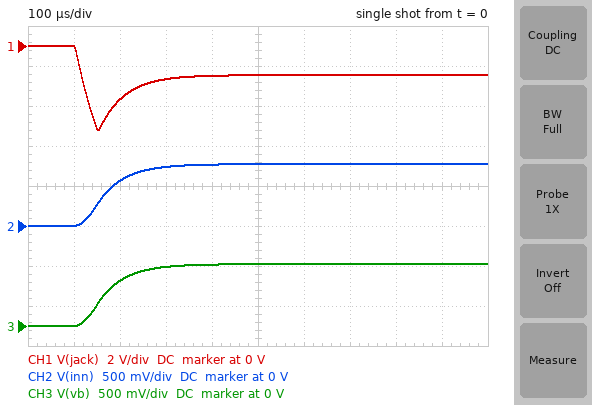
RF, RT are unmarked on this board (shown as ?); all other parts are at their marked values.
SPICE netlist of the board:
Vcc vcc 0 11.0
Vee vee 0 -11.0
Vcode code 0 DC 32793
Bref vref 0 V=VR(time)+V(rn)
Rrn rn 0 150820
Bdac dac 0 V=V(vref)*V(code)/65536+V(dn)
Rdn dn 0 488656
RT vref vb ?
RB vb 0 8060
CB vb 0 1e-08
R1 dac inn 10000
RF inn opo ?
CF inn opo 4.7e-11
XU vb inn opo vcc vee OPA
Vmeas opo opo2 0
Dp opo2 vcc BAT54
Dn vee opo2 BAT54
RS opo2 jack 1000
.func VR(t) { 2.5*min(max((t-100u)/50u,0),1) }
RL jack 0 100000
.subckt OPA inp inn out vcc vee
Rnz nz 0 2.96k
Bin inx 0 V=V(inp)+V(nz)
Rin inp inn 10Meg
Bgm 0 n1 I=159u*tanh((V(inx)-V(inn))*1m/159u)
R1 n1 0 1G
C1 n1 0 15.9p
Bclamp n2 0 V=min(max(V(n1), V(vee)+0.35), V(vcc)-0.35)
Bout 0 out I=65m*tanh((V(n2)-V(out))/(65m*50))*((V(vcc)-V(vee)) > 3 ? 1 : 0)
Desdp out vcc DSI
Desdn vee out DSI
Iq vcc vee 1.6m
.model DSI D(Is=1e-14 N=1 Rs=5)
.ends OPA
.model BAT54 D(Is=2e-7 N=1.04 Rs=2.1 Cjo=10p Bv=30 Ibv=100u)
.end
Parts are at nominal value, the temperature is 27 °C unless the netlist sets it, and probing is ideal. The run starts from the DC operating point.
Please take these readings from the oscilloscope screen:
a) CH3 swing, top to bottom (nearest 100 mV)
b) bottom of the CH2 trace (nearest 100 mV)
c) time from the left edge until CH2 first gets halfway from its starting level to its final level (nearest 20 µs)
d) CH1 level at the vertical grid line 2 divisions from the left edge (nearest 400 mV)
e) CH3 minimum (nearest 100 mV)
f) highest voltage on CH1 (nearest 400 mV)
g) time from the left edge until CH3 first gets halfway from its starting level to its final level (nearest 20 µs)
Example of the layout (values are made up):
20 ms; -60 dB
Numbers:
800 mV; 0 V; 160 µs; -2.8 V; 0 V; 0 V; 160 µs
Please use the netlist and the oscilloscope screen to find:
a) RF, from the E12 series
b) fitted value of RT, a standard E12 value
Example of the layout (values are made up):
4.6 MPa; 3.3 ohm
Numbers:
47 kΩ; 18 kΩ
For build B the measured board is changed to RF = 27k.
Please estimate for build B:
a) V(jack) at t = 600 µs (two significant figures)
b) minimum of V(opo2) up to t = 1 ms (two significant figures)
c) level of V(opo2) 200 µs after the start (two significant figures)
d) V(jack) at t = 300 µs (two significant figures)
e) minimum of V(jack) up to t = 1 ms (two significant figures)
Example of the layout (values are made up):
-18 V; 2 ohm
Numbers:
-510 mV; -2.4 V; -1.3 V; -640 mV; -2.3 V
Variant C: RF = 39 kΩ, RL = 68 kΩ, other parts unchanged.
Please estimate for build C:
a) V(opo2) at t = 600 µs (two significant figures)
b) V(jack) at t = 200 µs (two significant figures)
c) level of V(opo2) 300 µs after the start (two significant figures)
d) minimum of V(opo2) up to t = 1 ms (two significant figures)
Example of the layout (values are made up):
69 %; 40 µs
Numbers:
-1.1 V; -2.1 V; -1.3 V; -3.5 V
